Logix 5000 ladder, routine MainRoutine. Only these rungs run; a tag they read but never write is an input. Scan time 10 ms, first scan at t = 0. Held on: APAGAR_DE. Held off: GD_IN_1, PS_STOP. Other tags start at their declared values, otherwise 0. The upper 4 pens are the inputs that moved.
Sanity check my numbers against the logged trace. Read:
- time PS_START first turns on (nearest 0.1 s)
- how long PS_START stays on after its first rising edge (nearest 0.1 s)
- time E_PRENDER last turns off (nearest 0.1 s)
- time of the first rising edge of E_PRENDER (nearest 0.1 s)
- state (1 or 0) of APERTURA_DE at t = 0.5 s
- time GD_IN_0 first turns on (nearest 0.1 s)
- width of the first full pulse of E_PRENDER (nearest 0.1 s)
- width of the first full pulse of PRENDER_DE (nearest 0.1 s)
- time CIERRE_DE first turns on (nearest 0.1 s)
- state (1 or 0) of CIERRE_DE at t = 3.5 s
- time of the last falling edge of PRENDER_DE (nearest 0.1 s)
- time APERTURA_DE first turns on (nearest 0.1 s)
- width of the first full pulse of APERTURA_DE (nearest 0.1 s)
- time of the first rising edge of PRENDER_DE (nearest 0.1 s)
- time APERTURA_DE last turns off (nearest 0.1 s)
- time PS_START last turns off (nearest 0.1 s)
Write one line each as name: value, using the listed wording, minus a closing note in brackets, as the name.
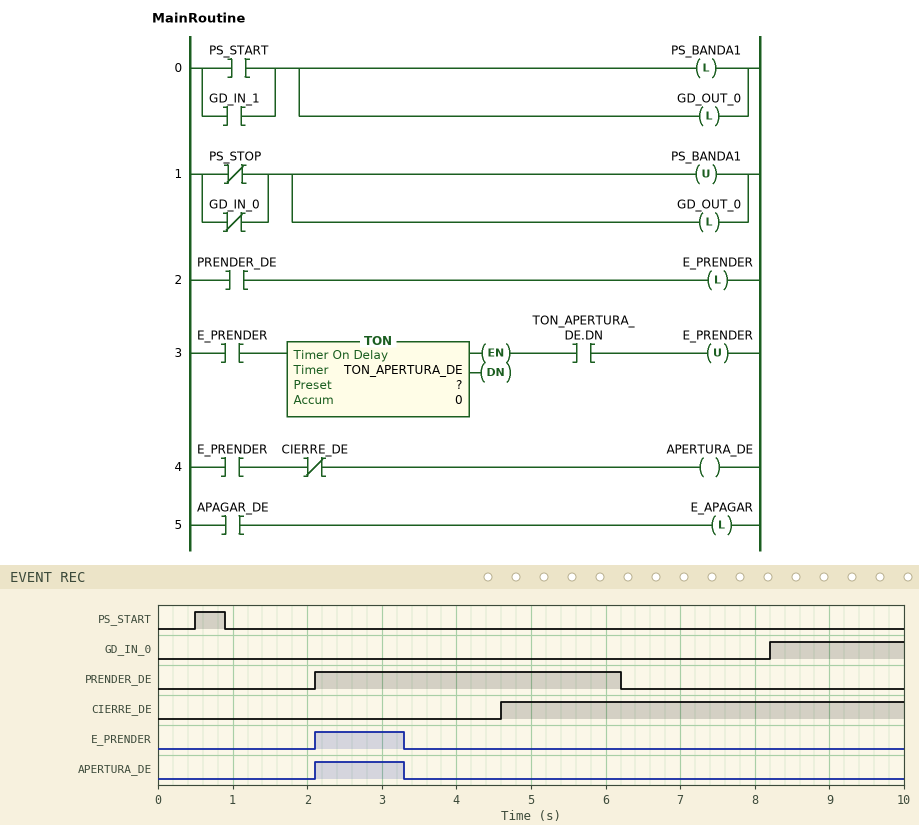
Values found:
time PS_START first turns on: 0.5 s
how long PS_START stays on after its first rising edge: 0.4 s
time E_PRENDER last turns off: 3.3 s
time of the first rising edge of E_PRENDER: 2.1 s
state (1 or 0) of APERTURA_DE at t = 0.5 s: 0
time GD_IN_0 first turns on: 8.2 s
width of the first full pulse of E_PRENDER: 1.2 s
width of the first full pulse of PRENDER_DE: 4.1 s
time CIERRE_DE first turns on: 4.6 s
state (1 or 0) of CIERRE_DE at t = 3.5 s: 0
time of the last falling edge of PRENDER_DE: 6.2 s
time APERTURA_DE first turns on: 2.1 s
width of the first full pulse of APERTURA_DE: 1.2 s
time of the first rising edge of PRENDER_DE: 2.1 s
time APERTURA_DE last turns off: 3.3 s
time PS_START last turns off: 0.9 s
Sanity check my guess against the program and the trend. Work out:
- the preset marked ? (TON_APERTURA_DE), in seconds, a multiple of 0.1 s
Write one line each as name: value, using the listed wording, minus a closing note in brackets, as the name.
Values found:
the preset marked ? (TON_APERTURA_DE), in seconds, a multiple of 0.1 s: 1.2 s
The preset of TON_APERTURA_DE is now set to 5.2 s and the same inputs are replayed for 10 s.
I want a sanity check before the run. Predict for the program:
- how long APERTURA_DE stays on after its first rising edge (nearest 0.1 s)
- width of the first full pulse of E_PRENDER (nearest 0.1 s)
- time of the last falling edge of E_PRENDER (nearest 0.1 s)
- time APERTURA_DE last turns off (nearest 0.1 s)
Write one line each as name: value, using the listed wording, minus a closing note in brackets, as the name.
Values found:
how long APERTURA_DE stays on after its first rising edge: 2.5 s
width of the first full pulse of E_PRENDER: 5.2 s
time of the last falling edge of E_PRENDER: 7.3 s
time APERTURA_DE last turns off: 4.6 s
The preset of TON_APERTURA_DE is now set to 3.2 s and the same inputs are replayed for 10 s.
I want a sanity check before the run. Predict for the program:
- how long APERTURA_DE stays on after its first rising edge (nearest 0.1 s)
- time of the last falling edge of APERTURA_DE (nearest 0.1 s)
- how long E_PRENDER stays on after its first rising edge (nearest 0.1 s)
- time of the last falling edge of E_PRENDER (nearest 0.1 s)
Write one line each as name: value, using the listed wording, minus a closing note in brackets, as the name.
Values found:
how long APERTURA_DE stays on after its first rising edge: 2.5 s
time of the last falling edge of APERTURA_DE: 4.6 s
how long E_PRENDER stays on after its first rising edge: 3.2 s
time of the last falling edge of E_PRENDER: 5.3 s
